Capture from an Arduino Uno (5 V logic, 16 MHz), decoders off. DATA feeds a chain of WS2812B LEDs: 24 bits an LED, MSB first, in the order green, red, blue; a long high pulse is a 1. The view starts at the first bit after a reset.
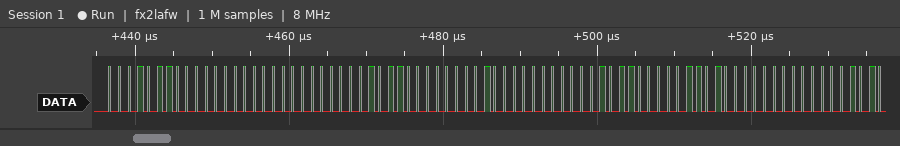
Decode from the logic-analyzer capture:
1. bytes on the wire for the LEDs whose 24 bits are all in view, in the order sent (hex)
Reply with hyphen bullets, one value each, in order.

- 16 00 00 16 01 00 16 0D 00
